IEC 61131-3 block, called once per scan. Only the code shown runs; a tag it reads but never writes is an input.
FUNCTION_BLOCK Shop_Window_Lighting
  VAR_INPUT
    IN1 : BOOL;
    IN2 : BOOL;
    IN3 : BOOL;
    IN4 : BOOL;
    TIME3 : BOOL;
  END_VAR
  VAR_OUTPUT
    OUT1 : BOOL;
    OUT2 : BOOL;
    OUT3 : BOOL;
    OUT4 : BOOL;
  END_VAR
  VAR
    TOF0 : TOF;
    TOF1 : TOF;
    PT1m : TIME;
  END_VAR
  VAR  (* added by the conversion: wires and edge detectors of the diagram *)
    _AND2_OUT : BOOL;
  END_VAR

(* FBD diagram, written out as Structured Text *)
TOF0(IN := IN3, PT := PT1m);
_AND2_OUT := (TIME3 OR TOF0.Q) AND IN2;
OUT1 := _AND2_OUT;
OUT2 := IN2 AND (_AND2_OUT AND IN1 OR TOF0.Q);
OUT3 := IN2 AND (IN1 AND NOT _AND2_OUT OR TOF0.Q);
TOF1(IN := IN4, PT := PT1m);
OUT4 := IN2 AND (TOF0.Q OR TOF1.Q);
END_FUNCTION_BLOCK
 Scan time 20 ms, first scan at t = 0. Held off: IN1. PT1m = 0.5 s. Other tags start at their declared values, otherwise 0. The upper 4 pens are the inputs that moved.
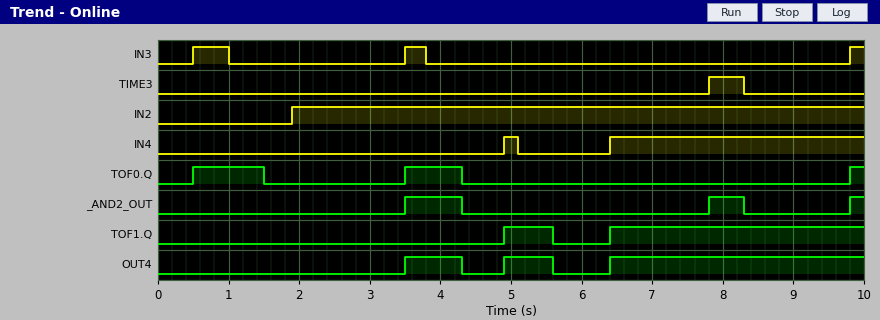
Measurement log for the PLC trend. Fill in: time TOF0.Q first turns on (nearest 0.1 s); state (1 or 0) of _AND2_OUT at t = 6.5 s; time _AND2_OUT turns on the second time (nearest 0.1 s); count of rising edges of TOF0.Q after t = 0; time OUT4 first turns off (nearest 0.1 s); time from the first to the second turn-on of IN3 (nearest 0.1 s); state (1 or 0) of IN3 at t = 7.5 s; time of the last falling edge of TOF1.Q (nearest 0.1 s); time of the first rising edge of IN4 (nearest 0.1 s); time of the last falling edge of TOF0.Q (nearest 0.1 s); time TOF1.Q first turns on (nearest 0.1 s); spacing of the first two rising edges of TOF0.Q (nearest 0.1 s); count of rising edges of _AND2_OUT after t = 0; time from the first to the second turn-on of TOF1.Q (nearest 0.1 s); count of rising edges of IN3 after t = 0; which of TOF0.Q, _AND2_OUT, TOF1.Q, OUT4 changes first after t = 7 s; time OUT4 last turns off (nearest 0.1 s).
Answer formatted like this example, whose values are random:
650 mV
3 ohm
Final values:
0.5 s
0
7.8 s
3
4.3 s
3.0 s
0
5.6 s
4.9 s
4.3 s
4.9 s
3.0 s
3
1.5 s
3
_AND2_OUT
5.6 s
